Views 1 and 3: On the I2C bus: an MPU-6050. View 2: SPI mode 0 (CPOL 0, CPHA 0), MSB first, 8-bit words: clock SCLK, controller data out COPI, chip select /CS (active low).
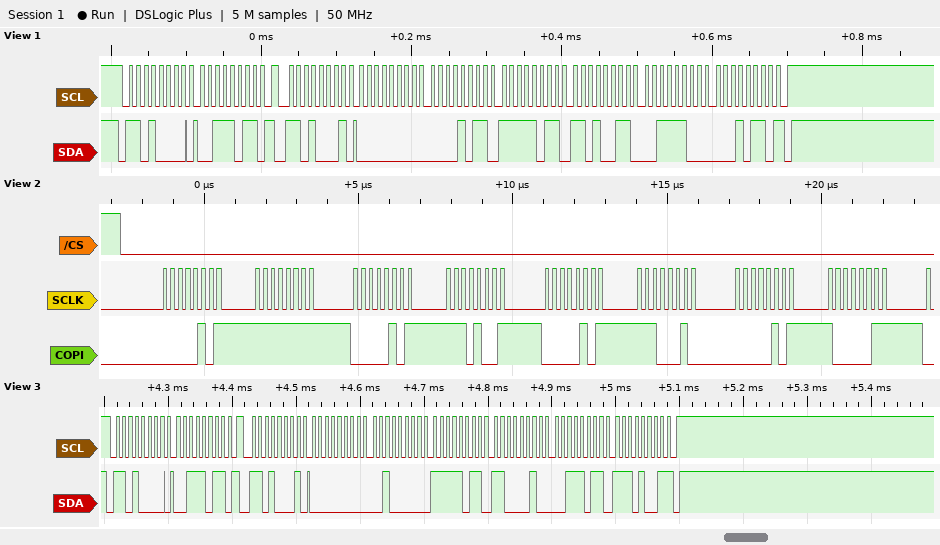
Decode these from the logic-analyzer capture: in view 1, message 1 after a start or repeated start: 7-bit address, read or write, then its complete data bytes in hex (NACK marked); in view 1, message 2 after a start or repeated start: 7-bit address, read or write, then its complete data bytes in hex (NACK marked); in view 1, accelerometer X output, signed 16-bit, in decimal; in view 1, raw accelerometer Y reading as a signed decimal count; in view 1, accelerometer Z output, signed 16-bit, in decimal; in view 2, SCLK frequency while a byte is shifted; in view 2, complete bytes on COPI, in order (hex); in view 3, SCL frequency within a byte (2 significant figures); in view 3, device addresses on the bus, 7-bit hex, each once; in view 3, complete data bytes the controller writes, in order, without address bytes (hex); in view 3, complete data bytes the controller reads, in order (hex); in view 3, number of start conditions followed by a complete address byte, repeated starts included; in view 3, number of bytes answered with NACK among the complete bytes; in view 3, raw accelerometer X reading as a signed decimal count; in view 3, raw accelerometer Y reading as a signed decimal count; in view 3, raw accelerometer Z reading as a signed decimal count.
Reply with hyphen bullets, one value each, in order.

- 0x68 write: 3B
- 0x68 read: 00 0B FB D3 3C 16 NACK
- 11
- -1069
- 15382
- 4 MHz
- 05 FF 05 E9 05 E2 05 83
- 100 kHz
- 0x68
- 3B
- 00 20 FB C2 3B E9
- 2
- 1
- 32
- -1086
- 15337
